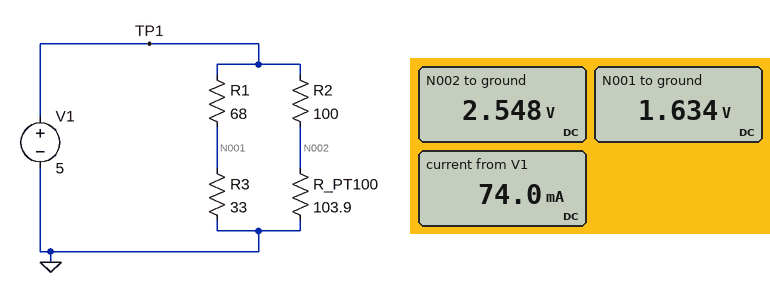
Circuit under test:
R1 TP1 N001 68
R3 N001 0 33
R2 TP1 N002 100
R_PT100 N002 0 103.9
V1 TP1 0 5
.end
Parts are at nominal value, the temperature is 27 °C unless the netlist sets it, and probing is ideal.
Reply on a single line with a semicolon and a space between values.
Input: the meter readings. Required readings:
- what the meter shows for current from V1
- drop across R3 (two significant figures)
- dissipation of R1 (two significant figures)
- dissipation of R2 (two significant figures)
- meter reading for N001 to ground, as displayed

74.0 mA; 1.6 V; 170 mW; 60 mW; 1.634 V
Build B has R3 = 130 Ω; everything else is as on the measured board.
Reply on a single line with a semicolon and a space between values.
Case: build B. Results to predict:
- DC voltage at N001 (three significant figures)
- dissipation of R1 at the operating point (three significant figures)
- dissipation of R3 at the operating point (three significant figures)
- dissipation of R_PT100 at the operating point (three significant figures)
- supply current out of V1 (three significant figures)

3.28 V; 43.4 mW; 82.9 mW; 62.5 mW; 49.8 mA
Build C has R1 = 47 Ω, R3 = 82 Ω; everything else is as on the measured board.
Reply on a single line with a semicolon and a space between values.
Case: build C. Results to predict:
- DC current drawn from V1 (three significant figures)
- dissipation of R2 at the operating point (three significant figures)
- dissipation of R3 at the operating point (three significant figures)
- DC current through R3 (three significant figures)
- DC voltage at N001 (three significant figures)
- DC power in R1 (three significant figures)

63.3 mA; 60.1 mW; 123 mW; 38.8 mA; 3.18 V; 70.6 mW
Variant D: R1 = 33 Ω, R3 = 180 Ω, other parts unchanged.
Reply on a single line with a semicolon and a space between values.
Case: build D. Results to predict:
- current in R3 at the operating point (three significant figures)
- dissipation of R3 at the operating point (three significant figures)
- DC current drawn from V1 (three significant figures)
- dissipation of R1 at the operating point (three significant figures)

23.5 mA; 99.2 mW; 48.0 mA; 18.2 mW
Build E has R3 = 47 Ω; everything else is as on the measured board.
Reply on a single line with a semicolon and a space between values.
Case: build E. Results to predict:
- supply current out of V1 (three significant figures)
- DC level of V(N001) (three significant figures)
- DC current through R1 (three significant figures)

68.0 mA; 2.04 V; 43.5 mA
